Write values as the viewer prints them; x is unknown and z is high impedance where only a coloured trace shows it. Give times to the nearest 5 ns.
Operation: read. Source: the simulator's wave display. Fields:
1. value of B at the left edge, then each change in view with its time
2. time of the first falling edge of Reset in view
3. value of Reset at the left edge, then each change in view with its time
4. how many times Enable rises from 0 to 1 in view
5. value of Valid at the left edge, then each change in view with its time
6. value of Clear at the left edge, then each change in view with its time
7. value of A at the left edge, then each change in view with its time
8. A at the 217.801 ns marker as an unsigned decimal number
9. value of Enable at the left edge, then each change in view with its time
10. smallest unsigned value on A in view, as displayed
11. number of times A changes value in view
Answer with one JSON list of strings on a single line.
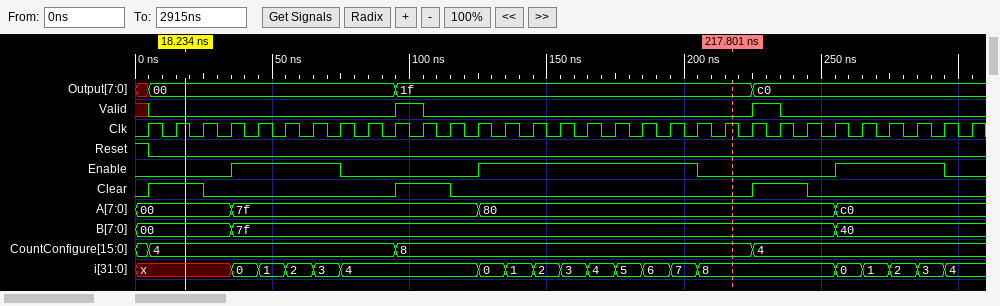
["00, 7f at 35 ns, 40 at 255 ns", "5 ns", "1, 0 at 5 ns", "3", "x, 0 at 5 ns, 1 at 95 ns, 0 at 105 ns, 1 at 225 ns, 0 at 235 ns", "0, 1 at 5 ns, 0 at 25 ns, 1 at 95 ns, 0 at 115 ns, 1 at 225 ns, 0 at 245 ns", "00, 7f at 35 ns, 80 at 125 ns, c0 at 255 ns", "128", "0, 1 at 35 ns, 0 at 75 ns, 1 at 125 ns, 0 at 205 ns, 1 at 255 ns, 0 at 295 ns", "00", "3"]
